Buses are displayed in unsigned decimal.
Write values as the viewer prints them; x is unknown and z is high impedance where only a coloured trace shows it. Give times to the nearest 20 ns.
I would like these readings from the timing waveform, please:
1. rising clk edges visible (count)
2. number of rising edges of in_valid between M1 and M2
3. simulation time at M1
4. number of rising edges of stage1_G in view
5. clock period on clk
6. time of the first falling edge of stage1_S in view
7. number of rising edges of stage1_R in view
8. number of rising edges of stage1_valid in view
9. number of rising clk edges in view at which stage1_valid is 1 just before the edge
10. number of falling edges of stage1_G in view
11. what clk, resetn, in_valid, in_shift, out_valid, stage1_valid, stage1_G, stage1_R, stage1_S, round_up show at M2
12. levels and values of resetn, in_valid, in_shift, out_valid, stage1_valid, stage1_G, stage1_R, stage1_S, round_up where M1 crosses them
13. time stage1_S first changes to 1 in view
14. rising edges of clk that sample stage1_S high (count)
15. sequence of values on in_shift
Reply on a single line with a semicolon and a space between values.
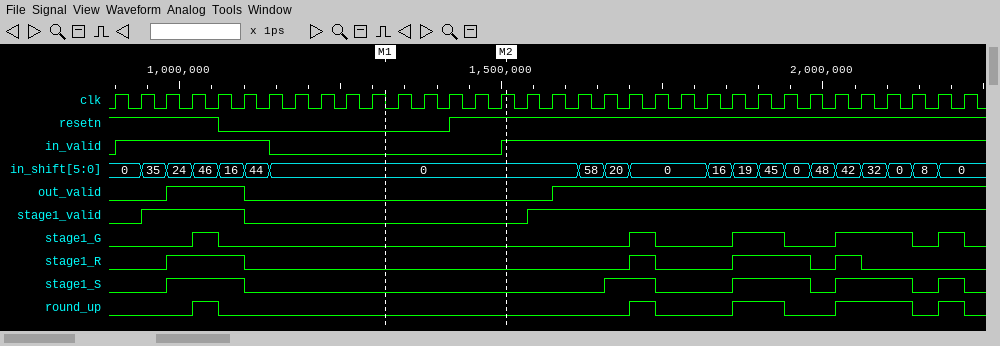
34; 1; 1320 ns; 5; 40 ns; 1100 ns; 4; 2; 21; 5; clk=1, resetn=1, in_valid=1, in_shift=0, out_valid=0, stage1_valid=0, stage1_G=0, stage1_R=0, stage1_S=0, round_up=0; resetn=0, in_valid=0, in_shift=0, out_valid=0, stage1_valid=0, stage1_G=0, stage1_R=0, stage1_S=0, round_up=0; 980 ns; 12; 0, 35, 24, 46, 16, 44, 0, 58, 20, 0, 16, 19, 45, 0, 48, 42, 32, 0, 8, 0
